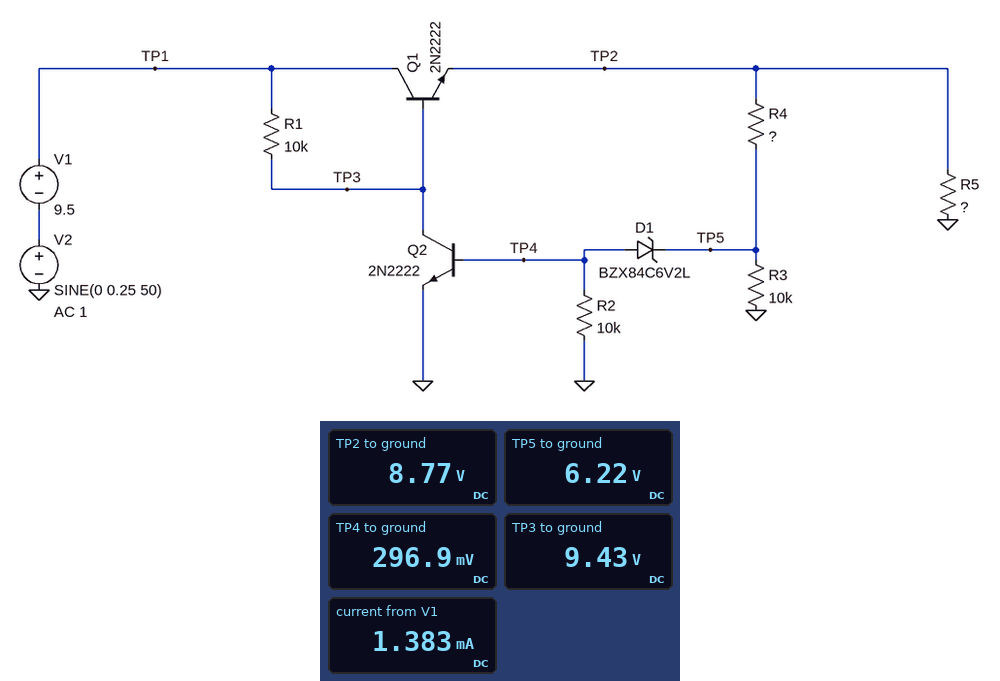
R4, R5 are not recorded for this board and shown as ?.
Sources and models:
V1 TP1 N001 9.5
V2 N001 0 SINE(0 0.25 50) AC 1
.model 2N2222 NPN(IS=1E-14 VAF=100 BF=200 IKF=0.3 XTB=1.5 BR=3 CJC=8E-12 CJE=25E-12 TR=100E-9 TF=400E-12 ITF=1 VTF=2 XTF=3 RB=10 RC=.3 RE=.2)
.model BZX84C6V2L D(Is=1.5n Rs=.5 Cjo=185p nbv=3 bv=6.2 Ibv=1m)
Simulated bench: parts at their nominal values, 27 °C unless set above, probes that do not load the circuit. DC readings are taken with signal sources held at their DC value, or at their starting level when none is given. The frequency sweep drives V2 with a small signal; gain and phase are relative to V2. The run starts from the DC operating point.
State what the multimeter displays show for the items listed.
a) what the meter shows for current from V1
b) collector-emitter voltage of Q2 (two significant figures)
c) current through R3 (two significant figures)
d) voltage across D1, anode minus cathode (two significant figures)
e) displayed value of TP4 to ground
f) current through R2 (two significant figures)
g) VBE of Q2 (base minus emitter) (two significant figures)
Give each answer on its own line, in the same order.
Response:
1.383 mA
9.4 V
620 µA
-5.9 V
296.9 mV
30 µA
300 mV
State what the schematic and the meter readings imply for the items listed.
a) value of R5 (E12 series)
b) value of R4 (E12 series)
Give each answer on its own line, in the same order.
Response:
12 kΩ
3.9 kΩ
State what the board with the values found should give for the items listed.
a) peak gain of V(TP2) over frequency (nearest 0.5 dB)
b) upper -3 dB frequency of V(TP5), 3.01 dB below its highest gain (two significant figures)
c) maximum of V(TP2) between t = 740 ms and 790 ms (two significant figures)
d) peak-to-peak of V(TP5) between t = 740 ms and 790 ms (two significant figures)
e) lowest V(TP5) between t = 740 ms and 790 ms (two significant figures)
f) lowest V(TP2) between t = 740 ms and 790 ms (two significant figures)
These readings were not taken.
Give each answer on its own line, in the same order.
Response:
0 dB
2.2 MHz
9.0 V
290 mV
6.1 V
8.5 V
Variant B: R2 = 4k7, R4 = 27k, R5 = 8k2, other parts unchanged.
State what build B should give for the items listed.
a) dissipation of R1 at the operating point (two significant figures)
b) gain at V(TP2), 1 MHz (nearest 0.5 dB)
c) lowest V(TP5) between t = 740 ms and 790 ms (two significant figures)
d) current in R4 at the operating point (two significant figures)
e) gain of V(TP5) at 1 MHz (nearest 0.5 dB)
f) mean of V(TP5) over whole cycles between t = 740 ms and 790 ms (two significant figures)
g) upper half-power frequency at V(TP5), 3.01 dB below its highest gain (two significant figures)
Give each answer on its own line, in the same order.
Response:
430 nW
-1.0 dB
2.3 V
240 µA
-19.5 dB
2.4 V
150 kHz
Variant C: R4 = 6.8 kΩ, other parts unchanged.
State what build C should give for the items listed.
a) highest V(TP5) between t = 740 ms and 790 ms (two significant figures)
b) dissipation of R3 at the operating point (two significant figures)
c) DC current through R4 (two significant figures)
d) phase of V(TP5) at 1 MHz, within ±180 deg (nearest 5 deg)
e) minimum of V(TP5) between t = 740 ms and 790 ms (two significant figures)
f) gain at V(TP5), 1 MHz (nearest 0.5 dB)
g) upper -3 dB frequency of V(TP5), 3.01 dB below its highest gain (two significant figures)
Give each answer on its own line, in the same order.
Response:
5.4 V
2.7 mW
520 µA
-25 deg
5.1 V
-7.5 dB
980 kHz
